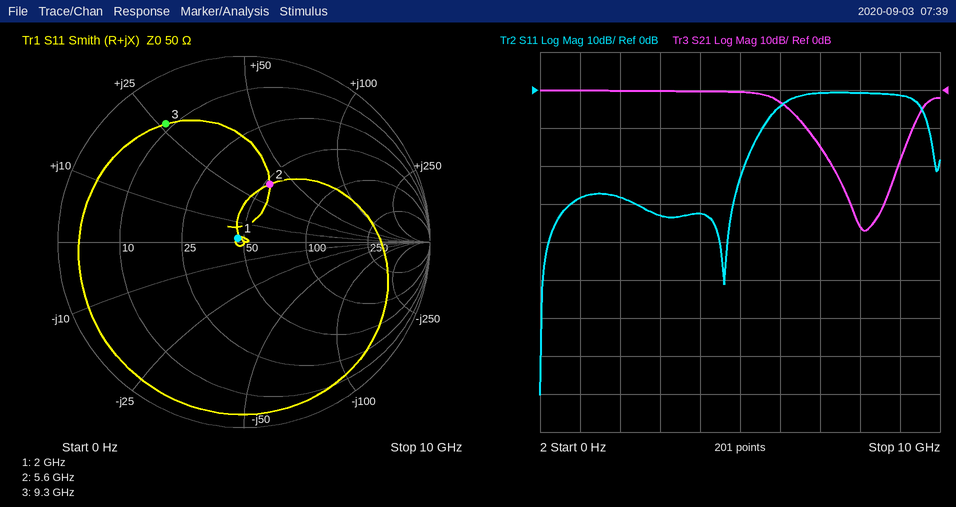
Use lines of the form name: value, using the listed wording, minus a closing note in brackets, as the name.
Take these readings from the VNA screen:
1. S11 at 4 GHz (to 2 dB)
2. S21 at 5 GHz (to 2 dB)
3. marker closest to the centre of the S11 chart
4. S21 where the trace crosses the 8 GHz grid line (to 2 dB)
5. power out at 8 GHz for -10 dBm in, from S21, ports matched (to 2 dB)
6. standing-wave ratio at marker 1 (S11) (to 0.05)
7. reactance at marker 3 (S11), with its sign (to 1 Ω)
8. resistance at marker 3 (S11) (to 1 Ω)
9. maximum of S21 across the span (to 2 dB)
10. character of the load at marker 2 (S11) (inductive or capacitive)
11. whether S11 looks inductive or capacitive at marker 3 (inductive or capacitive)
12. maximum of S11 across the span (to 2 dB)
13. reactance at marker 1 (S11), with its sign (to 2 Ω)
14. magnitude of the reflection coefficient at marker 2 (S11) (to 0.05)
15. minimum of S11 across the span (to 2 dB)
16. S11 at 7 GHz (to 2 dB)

S11 at 4 GHz: -32 dB
S21 at 5 GHz: 0 dB
marker closest to the centre of the S11 chart: marker 1
S21 where the trace crosses the 8 GHz grid line: -36 dB
power out at 8 GHz for -10 dBm in, from S21, ports matched: -46 dBm
standing-wave ratio at marker 1 (S11): 1.10
reactance at marker 3 (S11), with its sign: +26 Ω
resistance at marker 3 (S11): 9 Ω
maximum of S21 across the span: 0 dB
character of the load at marker 2 (S11): inductive
whether S11 looks inductive or capacitive at marker 3: inductive
maximum of S11 across the span: 0 dB
reactance at marker 1 (S11), with its sign: +2 Ω
magnitude of the reflection coefficient at marker 2 (S11): 0.35
minimum of S11 across the span: -80 dB
S11 at 7 GHz: 0 dB
